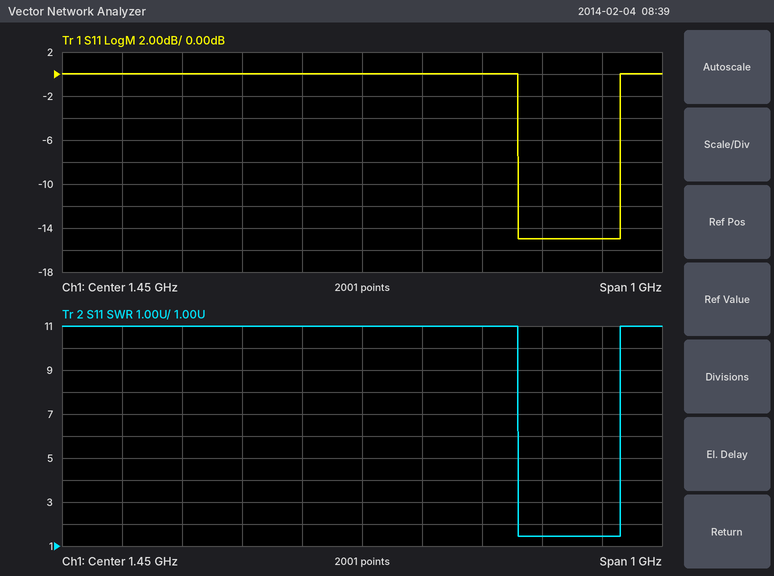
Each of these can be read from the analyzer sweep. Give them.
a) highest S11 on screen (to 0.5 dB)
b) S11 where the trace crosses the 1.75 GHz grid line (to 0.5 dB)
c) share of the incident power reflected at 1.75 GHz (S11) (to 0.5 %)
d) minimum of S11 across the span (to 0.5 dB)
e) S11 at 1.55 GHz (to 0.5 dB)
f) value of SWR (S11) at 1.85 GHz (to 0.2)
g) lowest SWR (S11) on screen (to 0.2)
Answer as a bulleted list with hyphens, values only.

- 0.0 dB
- -15.0 dB
- 3.0 %
- -15.0 dB
- 0.0 dB
- 1.4
- 1.4
